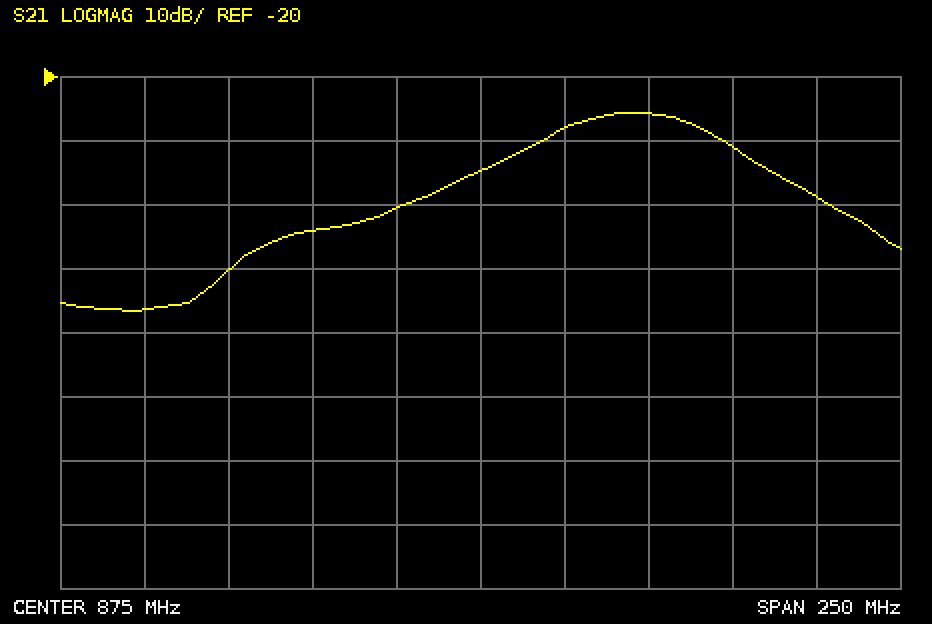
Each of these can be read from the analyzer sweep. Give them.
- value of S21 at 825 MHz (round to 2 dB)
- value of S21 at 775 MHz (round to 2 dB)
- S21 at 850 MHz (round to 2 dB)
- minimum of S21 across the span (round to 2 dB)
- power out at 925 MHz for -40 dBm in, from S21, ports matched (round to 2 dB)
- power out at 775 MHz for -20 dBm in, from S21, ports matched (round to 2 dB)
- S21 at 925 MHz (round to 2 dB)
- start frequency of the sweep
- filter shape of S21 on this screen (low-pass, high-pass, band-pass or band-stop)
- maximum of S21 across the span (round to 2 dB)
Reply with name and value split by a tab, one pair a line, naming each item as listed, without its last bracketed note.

value of S21 at 825 MHz	-44 dB
value of S21 at 775 MHz	-56 dB
S21 at 850 MHz	-40 dB
minimum of S21 across the span	-56 dB
power out at 925 MHz for -40 dBm in, from S21, ports matched	-66 dBm
power out at 775 MHz for -20 dBm in, from S21, ports matched	-76 dBm
S21 at 925 MHz	-26 dB
start frequency of the sweep	750 MHz
filter shape of S21 on this screen	band-pass
maximum of S21 across the span	-26 dB
